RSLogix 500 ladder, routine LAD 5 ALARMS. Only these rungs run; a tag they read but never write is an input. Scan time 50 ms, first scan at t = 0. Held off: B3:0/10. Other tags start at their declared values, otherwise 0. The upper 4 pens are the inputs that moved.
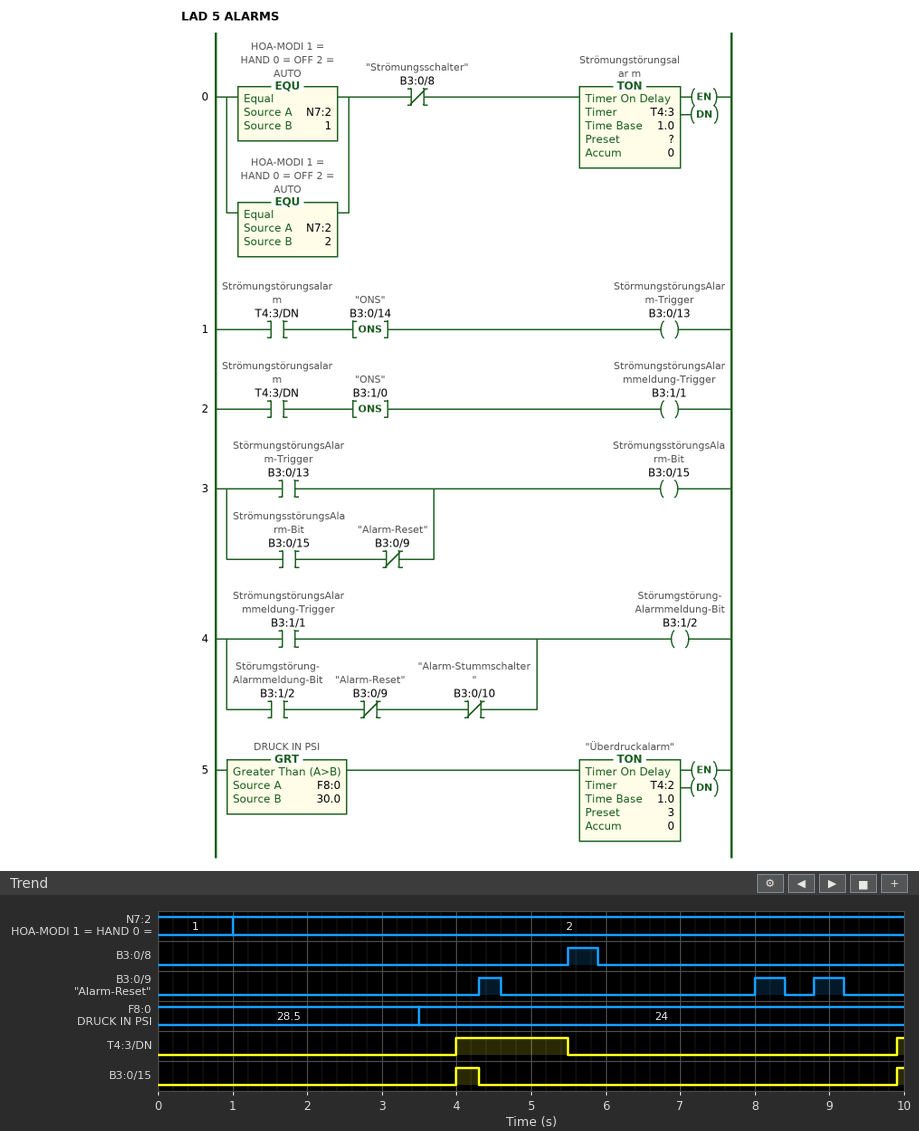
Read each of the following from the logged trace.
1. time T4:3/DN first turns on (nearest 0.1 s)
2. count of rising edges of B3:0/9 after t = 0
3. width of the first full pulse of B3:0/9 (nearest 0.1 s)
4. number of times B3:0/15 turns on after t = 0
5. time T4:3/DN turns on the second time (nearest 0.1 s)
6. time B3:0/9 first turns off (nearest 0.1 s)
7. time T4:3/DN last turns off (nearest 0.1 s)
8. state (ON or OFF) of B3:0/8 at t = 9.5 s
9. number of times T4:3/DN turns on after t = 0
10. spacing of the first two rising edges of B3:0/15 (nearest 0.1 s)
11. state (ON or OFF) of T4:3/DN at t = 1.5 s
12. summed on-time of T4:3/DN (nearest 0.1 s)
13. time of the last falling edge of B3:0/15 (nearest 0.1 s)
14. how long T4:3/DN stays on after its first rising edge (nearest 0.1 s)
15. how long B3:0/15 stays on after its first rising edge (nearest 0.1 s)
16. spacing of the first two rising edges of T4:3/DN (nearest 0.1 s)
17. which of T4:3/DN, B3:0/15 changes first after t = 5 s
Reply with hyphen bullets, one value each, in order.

- 4.0 s
- 3
- 0.3 s
- 2
- 9.9 s
- 4.6 s
- 5.5 s
- OFF
- 2
- 5.9 s
- OFF
- 1.6 s
- 4.3 s
- 1.5 s
- 0.3 s
- 5.9 s
- T4:3/DN
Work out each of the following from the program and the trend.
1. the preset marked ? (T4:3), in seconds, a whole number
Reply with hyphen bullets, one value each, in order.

- 4 s
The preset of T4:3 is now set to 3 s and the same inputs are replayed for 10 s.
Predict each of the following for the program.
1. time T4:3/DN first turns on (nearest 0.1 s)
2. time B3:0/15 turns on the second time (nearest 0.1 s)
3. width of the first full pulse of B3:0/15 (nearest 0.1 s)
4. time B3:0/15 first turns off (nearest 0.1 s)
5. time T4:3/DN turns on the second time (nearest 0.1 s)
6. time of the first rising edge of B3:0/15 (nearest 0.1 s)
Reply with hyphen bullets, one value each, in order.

- 3.0 s
- 8.9 s
- 1.3 s
- 4.3 s
- 8.9 s
- 3.0 s
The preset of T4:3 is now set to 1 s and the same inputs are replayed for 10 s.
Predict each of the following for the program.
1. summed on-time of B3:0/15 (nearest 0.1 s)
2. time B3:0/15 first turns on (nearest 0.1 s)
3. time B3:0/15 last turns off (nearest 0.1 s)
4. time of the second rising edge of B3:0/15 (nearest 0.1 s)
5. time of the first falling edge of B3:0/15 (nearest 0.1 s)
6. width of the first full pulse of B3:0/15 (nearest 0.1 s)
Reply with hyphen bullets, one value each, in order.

- 4.4 s
- 1.0 s
- 8.0 s
- 6.9 s
- 4.3 s
- 3.3 s
